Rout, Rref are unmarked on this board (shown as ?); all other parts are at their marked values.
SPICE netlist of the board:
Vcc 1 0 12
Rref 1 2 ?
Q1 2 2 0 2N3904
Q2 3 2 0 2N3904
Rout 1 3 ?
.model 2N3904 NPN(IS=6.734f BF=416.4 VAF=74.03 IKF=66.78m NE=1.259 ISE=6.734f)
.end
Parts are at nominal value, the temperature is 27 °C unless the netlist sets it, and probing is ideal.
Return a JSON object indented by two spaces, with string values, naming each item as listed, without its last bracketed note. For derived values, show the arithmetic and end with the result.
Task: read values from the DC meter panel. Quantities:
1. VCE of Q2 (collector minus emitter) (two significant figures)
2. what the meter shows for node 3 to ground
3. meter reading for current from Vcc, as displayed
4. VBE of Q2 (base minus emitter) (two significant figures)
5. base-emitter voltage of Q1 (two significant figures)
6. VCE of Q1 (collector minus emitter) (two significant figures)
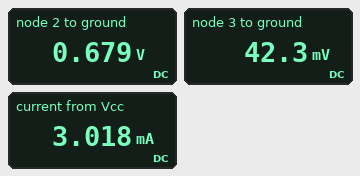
{
  "VCE of Q2 (collector minus emitter)": "42.3 mV = 42 mV",
  "what the meter shows for node 3 to ground": "42.3 mV",
  "meter reading for current from Vcc, as displayed": "3.018 mA",
  "VBE of Q2 (base minus emitter)": "679 mV = 680 mV",
  "base-emitter voltage of Q1": "679 mV = 680 mV",
  "VCE of Q1 (collector minus emitter)": "679 mV = 680 mV"
}
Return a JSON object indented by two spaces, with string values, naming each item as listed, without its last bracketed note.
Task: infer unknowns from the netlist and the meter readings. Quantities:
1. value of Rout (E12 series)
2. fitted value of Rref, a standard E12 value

{
  "value of Rout": "12 kΩ",
  "fitted value of Rref, a standard E12 value": "5.6 kΩ"
}
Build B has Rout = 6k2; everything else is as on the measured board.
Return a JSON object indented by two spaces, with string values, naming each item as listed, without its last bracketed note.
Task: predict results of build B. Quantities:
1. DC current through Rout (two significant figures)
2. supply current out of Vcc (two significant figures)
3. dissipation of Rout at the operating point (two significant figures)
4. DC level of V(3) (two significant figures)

{
  "DC current through Rout": "1.9 mA",
  "supply current out of Vcc": "3.9 mA",
  "dissipation of Rout at the operating point": "23 mW",
  "DC level of V(3)": "120 mV"
}
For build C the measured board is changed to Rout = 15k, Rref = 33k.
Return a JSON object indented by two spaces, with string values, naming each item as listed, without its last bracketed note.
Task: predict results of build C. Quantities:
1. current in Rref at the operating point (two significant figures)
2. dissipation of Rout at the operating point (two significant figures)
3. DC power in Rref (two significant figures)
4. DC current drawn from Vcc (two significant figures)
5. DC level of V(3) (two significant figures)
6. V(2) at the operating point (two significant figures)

{
  "current in Rref at the operating point": "340 µA",
  "dissipation of Rout at the operating point": "2.0 mW",
  "DC power in Rref": "3.9 mW",
  "DC current drawn from Vcc": "710 µA",
  "DC level of V(3)": "6.5 V",
  "V(2) at the operating point": "640 mV"
}
